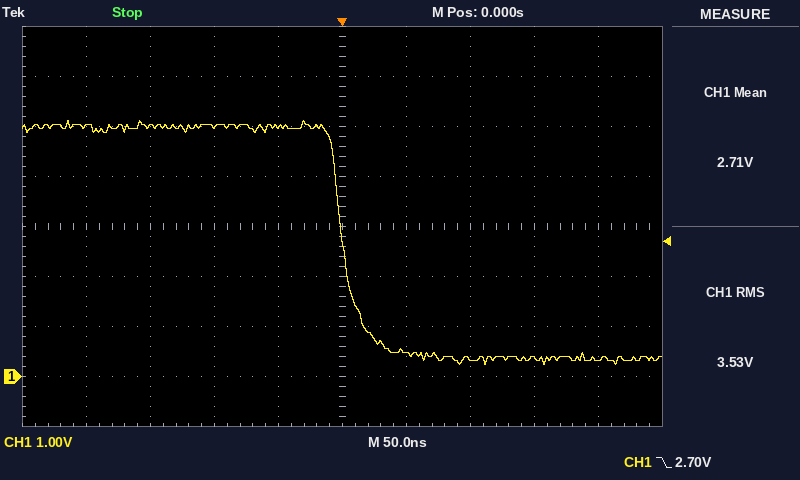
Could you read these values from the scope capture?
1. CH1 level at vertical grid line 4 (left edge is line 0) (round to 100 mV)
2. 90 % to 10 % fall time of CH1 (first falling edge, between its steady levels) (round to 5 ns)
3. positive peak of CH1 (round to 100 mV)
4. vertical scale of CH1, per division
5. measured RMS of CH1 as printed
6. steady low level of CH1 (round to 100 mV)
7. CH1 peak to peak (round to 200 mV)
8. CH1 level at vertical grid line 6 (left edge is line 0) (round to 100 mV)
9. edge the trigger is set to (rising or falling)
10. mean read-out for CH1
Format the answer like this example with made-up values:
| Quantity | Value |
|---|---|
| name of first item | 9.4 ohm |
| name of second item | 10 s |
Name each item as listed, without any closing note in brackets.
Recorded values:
| Quantity | Value |
|---|---|
| CH1 level at vertical grid line 4 (left edge is line 0) | 5.0 V |
| 90 % to 10 % fall time of CH1 (first falling edge, between its steady levels) | 30 ns |
| positive peak of CH1 | 5.1 V |
| vertical scale of CH1, per division | 1 V |
| measured RMS of CH1 as printed | 3.53 V |
| steady low level of CH1 | 400 mV |
| CH1 peak to peak | 4.8 V |
| CH1 level at vertical grid line 6 (left edge is line 0) | 500 mV |
| edge the trigger is set to | falling |
| mean read-out for CH1 | 2.71 V |
